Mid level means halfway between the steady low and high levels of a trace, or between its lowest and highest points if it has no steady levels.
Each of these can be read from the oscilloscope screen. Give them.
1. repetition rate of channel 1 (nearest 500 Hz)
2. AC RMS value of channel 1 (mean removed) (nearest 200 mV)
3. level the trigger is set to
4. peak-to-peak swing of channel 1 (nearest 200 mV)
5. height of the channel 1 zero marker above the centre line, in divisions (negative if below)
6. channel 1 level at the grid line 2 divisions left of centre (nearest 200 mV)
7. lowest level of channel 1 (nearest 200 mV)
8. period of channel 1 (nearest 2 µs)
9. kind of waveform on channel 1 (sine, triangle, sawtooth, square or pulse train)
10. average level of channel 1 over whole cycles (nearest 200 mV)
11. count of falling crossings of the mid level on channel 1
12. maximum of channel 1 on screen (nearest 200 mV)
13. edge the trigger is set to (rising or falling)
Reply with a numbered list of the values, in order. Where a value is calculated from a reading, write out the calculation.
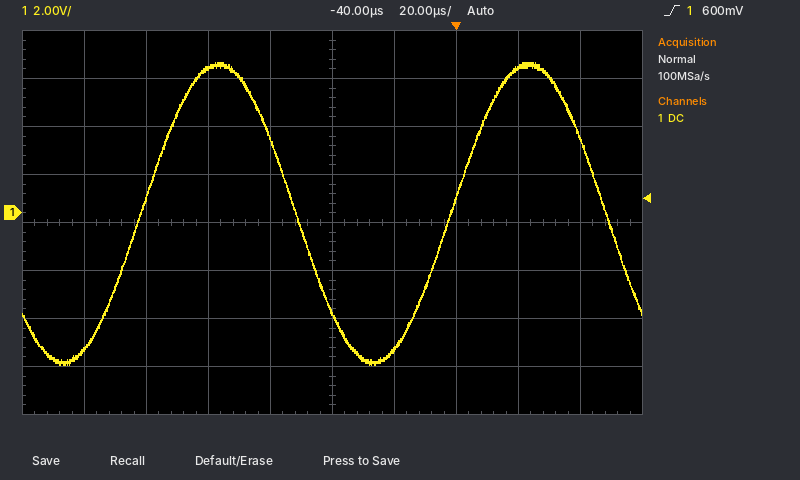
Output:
1. 1 / 100 µs ≈ 10.0 kHz
2. 12.6 V / (2√2) ≈ 4.4 V
3. 600 mV
4. 6.2 V − (-6.4 V) = 12.6 V
5. +0.2 div
6. 6.0 V
7. -6.4 V
8. 100 µs
9. sine
10. (6.2 V + (-6.4 V)) / 2 ≈ 0.0 V
11. 2
12. 6.2 V
13. rising
